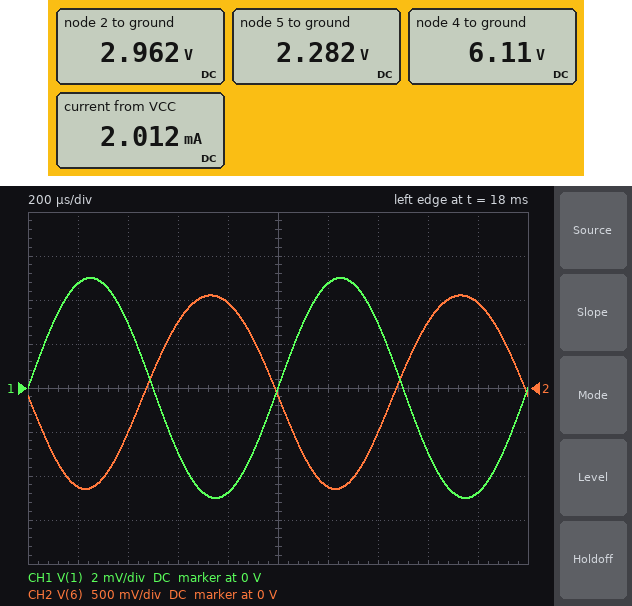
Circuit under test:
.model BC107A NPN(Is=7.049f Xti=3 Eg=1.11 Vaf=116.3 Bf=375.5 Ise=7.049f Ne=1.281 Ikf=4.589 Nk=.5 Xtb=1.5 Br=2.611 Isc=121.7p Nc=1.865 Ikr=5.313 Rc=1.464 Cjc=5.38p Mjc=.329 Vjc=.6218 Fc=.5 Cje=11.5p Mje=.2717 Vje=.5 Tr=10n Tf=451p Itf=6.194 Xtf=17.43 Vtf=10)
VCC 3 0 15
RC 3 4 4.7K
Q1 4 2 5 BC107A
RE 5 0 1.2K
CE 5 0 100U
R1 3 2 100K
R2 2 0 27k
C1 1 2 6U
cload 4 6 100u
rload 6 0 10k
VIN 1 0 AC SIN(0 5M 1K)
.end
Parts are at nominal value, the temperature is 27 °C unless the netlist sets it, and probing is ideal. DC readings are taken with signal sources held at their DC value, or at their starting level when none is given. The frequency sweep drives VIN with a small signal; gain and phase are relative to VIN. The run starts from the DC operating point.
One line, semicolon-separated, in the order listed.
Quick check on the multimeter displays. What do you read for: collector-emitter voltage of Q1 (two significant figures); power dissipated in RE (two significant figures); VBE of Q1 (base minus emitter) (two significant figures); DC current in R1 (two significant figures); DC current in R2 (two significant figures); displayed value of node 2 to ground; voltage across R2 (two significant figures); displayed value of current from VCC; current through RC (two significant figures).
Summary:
3.8 V; 4.3 mW; 680 mV; 120 µA; 110 µA; 2.962 V; 3.0 V; 2.012 mA; 1.9 mA
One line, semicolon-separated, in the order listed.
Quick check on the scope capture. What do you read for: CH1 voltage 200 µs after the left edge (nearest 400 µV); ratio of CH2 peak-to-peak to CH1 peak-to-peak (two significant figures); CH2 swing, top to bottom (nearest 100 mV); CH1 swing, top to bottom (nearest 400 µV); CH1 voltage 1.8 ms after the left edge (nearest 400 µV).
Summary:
4.8 mV; 220; 2.2 V; 10.0 mV; -4.8 mV
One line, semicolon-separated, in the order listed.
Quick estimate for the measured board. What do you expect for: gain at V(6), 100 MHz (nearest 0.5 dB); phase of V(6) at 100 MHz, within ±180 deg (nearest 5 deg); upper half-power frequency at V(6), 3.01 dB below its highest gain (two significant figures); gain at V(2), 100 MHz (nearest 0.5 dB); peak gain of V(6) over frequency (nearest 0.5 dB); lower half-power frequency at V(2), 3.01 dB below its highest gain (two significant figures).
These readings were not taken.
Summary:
31.5 dB; 100 deg; 18 MHz; 0 dB; 47.0 dB; 1.5 Hz
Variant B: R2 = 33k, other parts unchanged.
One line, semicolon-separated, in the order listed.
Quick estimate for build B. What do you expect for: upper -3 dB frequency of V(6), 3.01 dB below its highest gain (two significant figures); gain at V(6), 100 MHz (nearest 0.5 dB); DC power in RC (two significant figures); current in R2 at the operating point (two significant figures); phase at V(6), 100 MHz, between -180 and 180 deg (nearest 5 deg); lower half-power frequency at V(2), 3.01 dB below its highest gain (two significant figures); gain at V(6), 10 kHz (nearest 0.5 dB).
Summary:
13 MHz; 31.0 dB; 24 mW; 100 µA; 95 deg; 1.3 Hz; 48.5 dB
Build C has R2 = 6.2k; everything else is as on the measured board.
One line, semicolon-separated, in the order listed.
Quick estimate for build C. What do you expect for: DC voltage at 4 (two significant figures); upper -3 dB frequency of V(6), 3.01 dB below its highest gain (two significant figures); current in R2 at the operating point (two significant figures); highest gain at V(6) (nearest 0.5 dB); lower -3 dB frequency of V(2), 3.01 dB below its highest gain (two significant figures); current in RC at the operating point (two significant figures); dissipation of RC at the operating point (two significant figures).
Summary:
14 V; 26 MHz; 140 µA; 28.0 dB; 5.2 Hz; 200 µA; 200 µW
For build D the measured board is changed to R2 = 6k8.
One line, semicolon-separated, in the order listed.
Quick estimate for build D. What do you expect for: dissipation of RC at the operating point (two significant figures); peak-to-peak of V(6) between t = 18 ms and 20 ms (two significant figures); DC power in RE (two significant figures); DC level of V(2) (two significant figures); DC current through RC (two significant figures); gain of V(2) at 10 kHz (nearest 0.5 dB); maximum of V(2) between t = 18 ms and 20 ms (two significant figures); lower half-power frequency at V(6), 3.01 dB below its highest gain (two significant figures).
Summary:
320 µW; 320 mV; 84 µW; 940 mV; 260 µA; 0 dB; 950 mV; 20 Hz
